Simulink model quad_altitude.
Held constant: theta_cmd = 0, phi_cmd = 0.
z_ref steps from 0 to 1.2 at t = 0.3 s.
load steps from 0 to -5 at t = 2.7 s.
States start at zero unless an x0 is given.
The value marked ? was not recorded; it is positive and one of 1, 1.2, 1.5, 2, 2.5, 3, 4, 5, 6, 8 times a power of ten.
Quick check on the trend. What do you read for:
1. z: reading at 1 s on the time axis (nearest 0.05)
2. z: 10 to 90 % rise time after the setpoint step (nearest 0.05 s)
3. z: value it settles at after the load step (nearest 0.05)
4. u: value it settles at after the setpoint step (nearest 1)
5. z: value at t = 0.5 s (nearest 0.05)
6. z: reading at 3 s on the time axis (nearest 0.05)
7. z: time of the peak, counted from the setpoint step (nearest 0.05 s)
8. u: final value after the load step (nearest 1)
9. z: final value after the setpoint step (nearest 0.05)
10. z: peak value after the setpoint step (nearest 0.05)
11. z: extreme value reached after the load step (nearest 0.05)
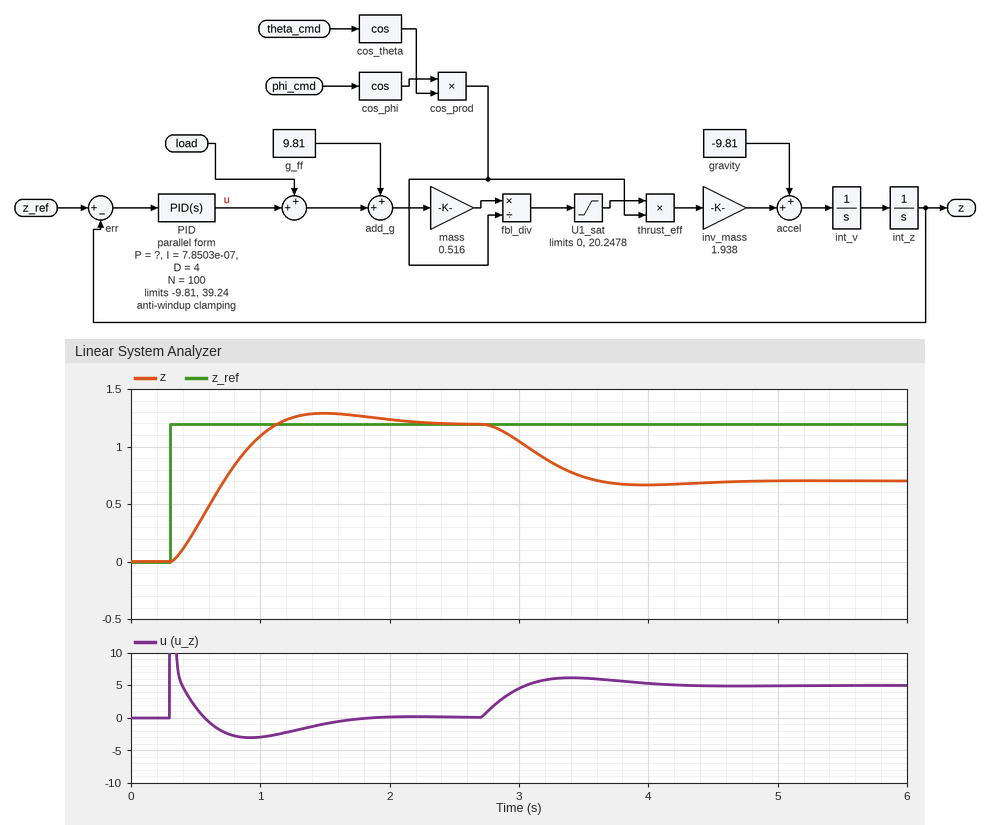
1.10
0.60 s
0.70
0
0.30
1.05
1.20 s
5
1.20
1.30
0.65
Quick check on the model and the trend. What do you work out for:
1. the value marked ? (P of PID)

10
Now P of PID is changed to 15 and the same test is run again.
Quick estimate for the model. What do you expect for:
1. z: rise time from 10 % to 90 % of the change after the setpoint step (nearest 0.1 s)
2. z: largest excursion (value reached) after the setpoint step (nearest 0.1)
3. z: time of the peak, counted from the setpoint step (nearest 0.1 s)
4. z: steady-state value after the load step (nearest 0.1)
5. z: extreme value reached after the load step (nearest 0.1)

0.4 s
1.4
0.9 s
0.9
0.8
